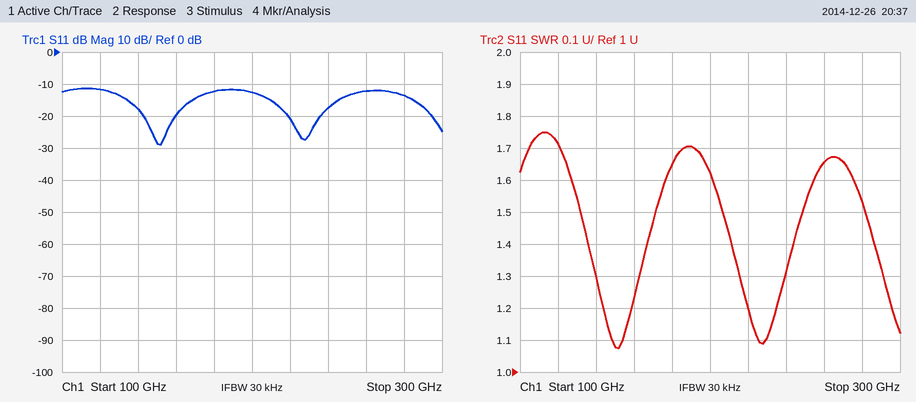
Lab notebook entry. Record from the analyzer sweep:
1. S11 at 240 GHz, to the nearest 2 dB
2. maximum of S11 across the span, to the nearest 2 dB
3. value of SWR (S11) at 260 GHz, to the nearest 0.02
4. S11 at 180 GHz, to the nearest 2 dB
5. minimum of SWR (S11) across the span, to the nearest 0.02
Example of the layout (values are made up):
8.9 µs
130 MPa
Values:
-18 dB
-12 dB
1.66
-12 dB
1.08
